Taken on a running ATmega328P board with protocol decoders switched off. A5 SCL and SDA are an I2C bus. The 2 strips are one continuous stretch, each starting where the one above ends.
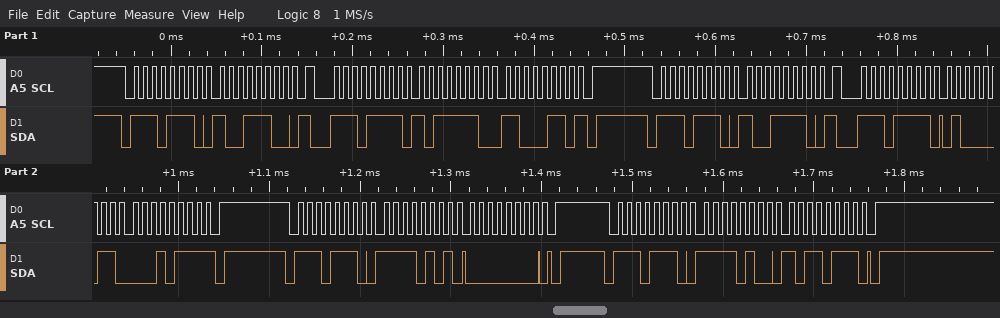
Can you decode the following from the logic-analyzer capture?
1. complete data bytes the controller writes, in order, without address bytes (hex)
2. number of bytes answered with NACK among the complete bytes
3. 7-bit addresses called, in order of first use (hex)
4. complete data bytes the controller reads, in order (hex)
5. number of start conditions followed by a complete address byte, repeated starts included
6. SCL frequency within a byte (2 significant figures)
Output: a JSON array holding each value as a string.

["9C 9E F5 00 F4 B7", "2", "0x77", "BE C6 43 17", "6", "100 kHz"]
